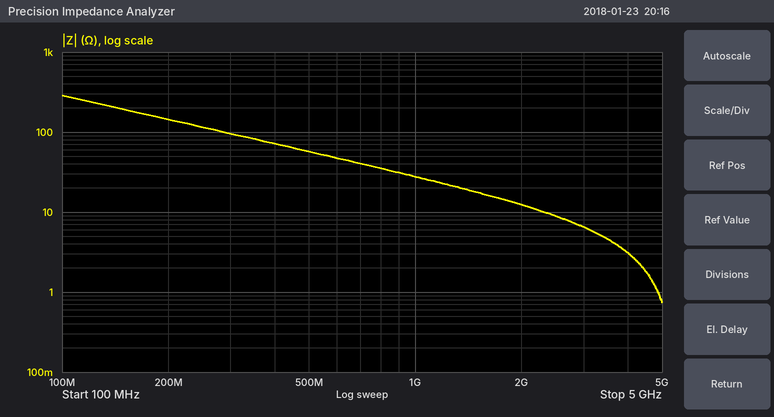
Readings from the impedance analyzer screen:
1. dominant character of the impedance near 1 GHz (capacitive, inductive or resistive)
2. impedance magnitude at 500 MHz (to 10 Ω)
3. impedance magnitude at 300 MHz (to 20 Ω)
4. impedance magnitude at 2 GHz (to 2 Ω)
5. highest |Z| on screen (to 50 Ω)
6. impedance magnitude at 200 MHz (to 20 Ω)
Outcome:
capacitive
60 Ω
100 Ω
12 Ω
300 Ω
140 Ω
